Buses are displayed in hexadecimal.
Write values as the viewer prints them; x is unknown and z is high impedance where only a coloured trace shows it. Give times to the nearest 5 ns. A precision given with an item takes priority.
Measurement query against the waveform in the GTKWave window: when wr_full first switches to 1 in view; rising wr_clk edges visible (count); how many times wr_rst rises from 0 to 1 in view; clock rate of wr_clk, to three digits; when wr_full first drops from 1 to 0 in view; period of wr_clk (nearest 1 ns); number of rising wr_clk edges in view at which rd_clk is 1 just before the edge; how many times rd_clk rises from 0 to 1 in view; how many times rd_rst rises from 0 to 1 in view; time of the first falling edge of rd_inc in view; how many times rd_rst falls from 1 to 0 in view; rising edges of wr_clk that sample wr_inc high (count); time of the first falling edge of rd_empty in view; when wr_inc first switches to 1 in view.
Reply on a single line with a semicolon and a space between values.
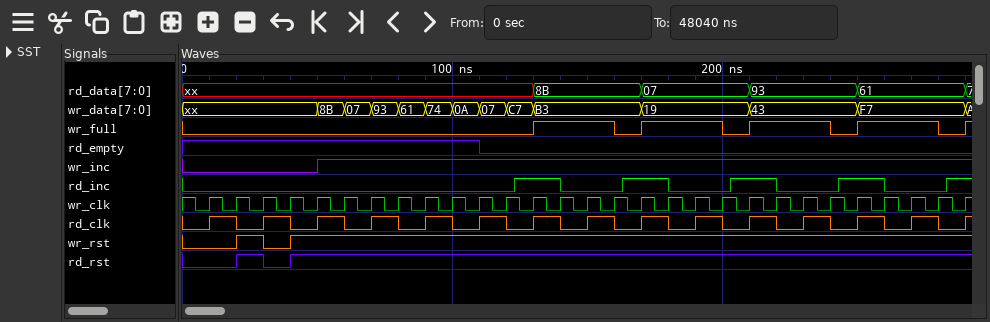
130 ns; 29; 2; 100 MHz; 160 ns; 10 ns; 14; 15; 2; 140 ns; 1; 24; 110 ns; 50 ns
